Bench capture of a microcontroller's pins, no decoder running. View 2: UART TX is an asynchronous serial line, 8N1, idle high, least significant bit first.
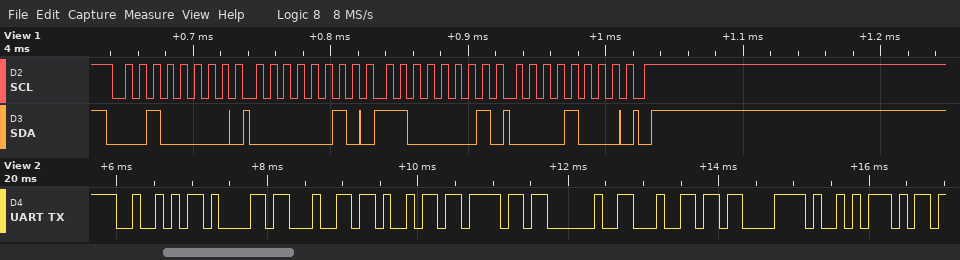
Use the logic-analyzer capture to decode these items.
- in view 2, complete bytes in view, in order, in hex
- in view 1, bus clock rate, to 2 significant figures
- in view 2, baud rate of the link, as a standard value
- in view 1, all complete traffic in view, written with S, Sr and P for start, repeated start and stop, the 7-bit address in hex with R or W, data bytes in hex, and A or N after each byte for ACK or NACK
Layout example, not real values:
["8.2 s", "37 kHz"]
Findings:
["0x52 0x61 0x64 0x69 0x6F 0x20 0x64 0xC3 0xA9", "100 kHz", "9600 baud", "S 10W A 02 A C1 A 08 A P"]
